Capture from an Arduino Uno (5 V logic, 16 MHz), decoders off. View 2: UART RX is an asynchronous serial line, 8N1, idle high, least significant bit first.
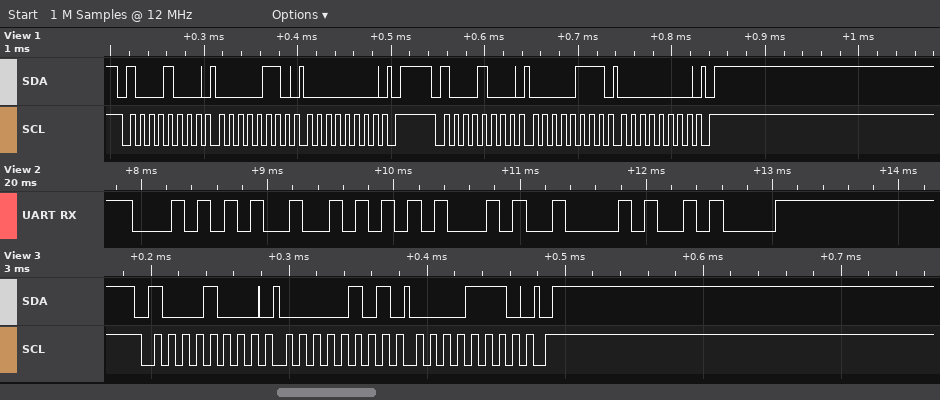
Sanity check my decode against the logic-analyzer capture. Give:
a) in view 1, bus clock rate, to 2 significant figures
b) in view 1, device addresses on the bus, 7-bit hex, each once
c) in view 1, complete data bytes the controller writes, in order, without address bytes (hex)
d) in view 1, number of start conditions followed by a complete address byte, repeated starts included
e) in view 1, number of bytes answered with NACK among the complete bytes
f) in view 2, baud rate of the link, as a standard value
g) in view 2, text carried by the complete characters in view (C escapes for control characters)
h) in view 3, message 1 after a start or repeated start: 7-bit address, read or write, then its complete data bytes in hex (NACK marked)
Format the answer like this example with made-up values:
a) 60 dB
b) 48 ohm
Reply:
a) 100 kHz
b) 0x44
c) 06 00 07 00
d) 2
e) 0
f) 9600 baud
g) "TREB\n"
h) 0x44 write: 05 0E
